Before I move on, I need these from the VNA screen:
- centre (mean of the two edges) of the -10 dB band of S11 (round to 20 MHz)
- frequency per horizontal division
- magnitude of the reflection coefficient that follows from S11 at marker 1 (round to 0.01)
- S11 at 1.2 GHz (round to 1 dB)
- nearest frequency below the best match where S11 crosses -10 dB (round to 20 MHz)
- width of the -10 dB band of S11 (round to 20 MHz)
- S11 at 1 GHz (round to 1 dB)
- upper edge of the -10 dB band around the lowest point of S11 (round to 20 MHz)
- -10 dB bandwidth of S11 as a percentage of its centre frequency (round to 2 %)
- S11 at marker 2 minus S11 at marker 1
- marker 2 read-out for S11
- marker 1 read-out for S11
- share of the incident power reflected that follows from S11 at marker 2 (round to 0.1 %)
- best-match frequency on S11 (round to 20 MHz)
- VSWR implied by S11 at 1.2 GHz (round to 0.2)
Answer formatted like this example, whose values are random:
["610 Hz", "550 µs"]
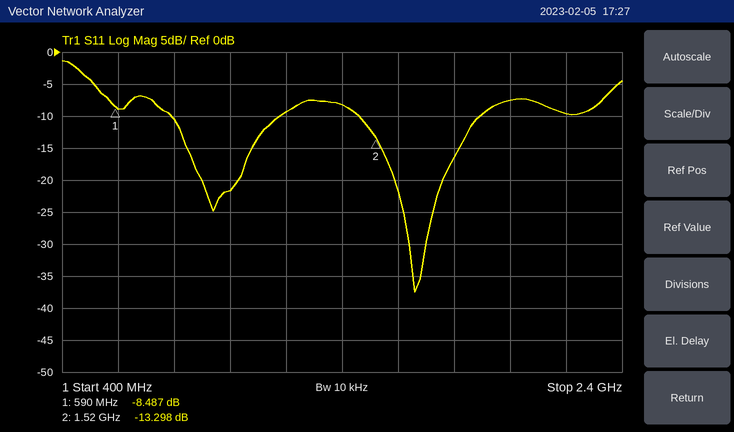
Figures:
["1.68 GHz", "200 MHz", "0.38", "-9 dB", "1.46 GHz", "440 MHz", "-22 dB", "1.90 GHz", "26 %", "-4.811 dB", "-13.298 dB", "-8.487 dB", "4.7 %", "1.66 GHz", "2.0"]
